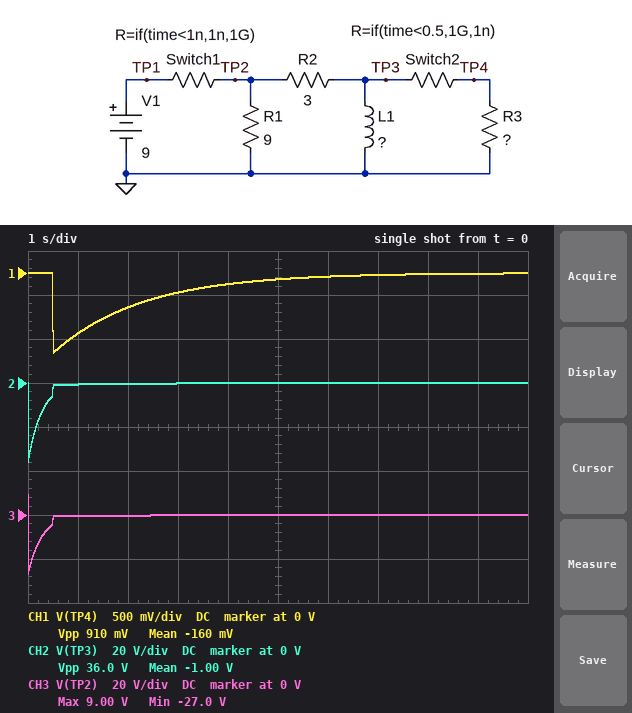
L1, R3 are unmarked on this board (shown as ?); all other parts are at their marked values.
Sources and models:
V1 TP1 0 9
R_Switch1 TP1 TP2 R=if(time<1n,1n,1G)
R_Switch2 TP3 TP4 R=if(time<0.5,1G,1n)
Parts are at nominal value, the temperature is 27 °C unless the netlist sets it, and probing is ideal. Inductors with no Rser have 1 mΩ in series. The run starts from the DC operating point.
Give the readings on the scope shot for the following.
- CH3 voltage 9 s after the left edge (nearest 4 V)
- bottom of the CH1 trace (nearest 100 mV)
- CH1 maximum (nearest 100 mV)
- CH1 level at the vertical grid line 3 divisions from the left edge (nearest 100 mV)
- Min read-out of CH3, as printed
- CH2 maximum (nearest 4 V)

0 V
-900 mV
0 V
-200 mV
-27.0 V
0 V
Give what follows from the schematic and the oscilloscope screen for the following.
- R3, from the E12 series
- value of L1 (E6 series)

2.2 Ω
3.3 H
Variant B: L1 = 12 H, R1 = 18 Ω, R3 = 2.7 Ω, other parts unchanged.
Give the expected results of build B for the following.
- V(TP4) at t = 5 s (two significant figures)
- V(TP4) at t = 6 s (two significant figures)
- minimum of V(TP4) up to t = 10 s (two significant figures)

-1.2 V
-1.0 V
-3.0 V
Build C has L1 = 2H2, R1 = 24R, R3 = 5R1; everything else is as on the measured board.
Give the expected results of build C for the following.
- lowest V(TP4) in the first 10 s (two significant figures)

-28 mV
